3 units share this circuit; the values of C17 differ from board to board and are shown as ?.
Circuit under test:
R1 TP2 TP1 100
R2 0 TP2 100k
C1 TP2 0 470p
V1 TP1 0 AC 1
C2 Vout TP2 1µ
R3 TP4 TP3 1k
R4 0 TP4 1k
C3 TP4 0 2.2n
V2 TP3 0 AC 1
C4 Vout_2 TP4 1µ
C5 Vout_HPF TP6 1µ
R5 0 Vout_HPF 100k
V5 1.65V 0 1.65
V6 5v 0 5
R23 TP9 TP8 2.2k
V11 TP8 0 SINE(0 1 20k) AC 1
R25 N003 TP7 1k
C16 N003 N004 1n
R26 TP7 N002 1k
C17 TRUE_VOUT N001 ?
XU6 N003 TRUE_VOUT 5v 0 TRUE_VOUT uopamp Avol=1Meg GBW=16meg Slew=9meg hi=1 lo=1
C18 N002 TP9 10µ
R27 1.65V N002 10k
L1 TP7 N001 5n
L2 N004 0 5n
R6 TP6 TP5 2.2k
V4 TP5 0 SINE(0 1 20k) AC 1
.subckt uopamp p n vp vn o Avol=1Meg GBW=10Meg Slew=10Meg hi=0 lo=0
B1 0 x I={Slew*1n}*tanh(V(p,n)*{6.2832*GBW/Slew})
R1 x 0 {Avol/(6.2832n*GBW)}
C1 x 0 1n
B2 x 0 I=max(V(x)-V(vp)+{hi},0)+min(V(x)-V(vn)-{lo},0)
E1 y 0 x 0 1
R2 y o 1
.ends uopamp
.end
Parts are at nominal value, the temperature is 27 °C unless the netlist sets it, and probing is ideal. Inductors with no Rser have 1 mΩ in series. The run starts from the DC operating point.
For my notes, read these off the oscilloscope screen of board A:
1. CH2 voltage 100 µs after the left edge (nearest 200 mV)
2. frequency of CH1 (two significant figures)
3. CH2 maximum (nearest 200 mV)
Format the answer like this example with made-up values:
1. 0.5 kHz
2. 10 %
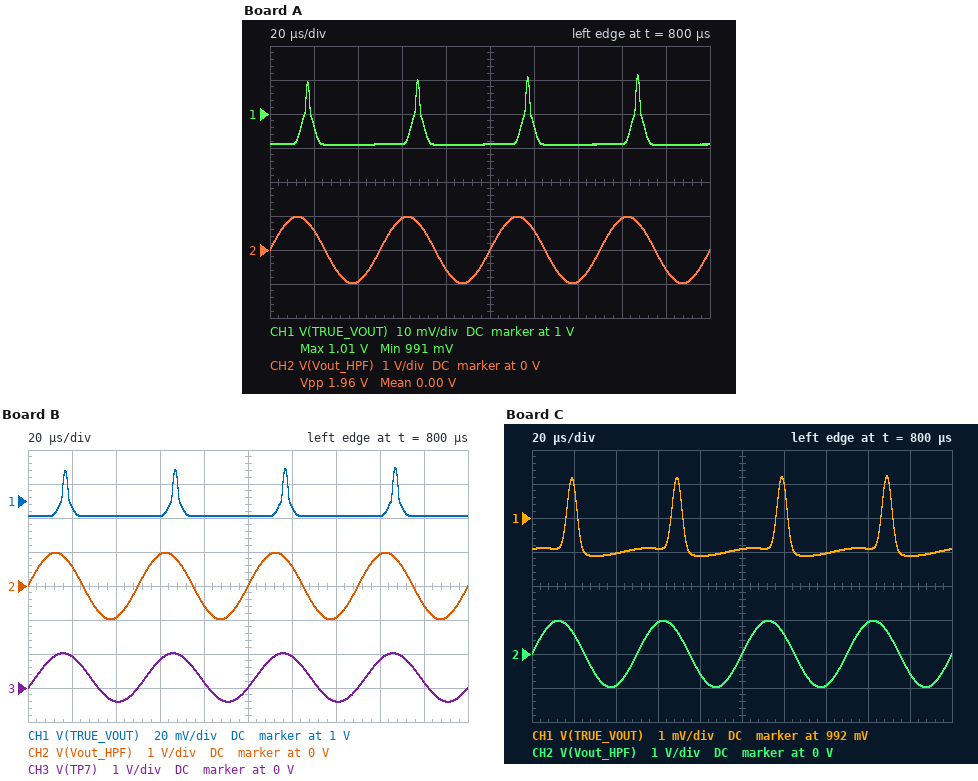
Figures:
1. 0 V
2. 20 kHz
3. 1.0 V
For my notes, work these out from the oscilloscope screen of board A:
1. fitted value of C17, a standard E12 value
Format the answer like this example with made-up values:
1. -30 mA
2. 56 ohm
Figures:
1. 470 pF
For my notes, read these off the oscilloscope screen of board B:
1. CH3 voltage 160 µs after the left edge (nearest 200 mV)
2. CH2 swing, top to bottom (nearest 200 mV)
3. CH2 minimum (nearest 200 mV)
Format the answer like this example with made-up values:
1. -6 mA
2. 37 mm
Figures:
1. 800 mV
2. 2.0 V
3. -1.0 V
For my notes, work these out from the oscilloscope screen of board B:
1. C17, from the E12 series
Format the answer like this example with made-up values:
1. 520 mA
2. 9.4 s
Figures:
1. 390 pF
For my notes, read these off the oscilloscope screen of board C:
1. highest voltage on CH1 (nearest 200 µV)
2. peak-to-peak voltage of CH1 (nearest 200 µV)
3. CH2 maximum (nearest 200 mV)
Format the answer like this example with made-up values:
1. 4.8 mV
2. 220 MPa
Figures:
1. 993.2 mV
2. 2.4 mV
3. 1.0 V
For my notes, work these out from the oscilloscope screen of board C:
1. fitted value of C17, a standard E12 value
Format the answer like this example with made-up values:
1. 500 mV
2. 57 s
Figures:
1. 1.5 nF
